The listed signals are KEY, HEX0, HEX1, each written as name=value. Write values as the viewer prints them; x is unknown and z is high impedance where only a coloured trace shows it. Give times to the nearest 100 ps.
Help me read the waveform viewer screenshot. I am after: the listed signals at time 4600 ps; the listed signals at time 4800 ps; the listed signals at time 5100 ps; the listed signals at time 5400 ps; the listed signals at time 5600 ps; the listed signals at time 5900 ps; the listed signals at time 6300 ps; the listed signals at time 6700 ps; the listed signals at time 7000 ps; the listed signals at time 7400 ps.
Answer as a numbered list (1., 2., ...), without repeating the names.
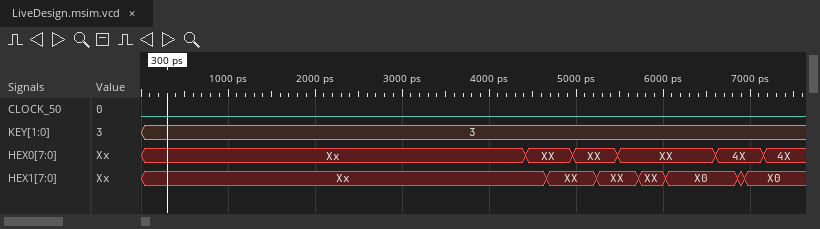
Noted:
1. KEY=3, HEX0=XX, HEX1=Xx
2. KEY=3, HEX0=XX, HEX1=XX
3. KEY=3, HEX0=XX, HEX1=XX
4. KEY=3, HEX0=XX, HEX1=XX
5. KEY=3, HEX0=XX, HEX1=XX
6. KEY=3, HEX0=XX, HEX1=XX
7. KEY=3, HEX0=XX, HEX1=X0
8. KEY=3, HEX0=4X, HEX1=X0
9. KEY=3, HEX0=4X, HEX1=X0
10. KEY=3, HEX0=4X, HEX1=X0
